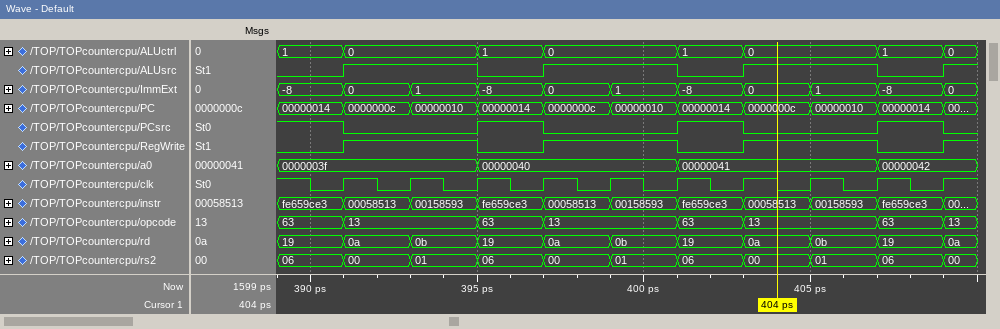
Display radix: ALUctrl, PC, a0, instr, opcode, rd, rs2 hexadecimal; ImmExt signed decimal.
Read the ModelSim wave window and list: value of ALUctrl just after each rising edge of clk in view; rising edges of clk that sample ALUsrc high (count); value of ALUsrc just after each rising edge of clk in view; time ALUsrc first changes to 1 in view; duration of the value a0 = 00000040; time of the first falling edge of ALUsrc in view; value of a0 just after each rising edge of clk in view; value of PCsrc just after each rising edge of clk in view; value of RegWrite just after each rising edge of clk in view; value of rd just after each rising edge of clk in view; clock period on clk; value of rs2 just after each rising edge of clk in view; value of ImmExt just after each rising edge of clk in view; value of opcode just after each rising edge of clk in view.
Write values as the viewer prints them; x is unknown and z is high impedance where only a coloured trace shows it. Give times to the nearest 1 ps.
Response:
0, 0, 1, 0, 0, 1, 0, 0, 1, 0
6
1 1 0 1 1 0 1 1 0 1
391 ps
6 ps
395 ps
0000003f, 0000003f, 00000040, 00000040, 00000040, 00000041, 00000041, 00000041, 00000042, 00000042
0 0 1 0 0 1 0 0 1 0
1 1 0 1 1 0 1 1 0 1
0a, 0b, 19, 0a, 0b, 19, 0a, 0b, 19, 0a
2 ps
00, 01, 06, 00, 01, 06, 00, 01, 06, 00
0, 1, -8, 0, 1, -8, 0, 1, -8, 0
13, 13, 63, 13, 13, 63, 13, 13, 63, 13
